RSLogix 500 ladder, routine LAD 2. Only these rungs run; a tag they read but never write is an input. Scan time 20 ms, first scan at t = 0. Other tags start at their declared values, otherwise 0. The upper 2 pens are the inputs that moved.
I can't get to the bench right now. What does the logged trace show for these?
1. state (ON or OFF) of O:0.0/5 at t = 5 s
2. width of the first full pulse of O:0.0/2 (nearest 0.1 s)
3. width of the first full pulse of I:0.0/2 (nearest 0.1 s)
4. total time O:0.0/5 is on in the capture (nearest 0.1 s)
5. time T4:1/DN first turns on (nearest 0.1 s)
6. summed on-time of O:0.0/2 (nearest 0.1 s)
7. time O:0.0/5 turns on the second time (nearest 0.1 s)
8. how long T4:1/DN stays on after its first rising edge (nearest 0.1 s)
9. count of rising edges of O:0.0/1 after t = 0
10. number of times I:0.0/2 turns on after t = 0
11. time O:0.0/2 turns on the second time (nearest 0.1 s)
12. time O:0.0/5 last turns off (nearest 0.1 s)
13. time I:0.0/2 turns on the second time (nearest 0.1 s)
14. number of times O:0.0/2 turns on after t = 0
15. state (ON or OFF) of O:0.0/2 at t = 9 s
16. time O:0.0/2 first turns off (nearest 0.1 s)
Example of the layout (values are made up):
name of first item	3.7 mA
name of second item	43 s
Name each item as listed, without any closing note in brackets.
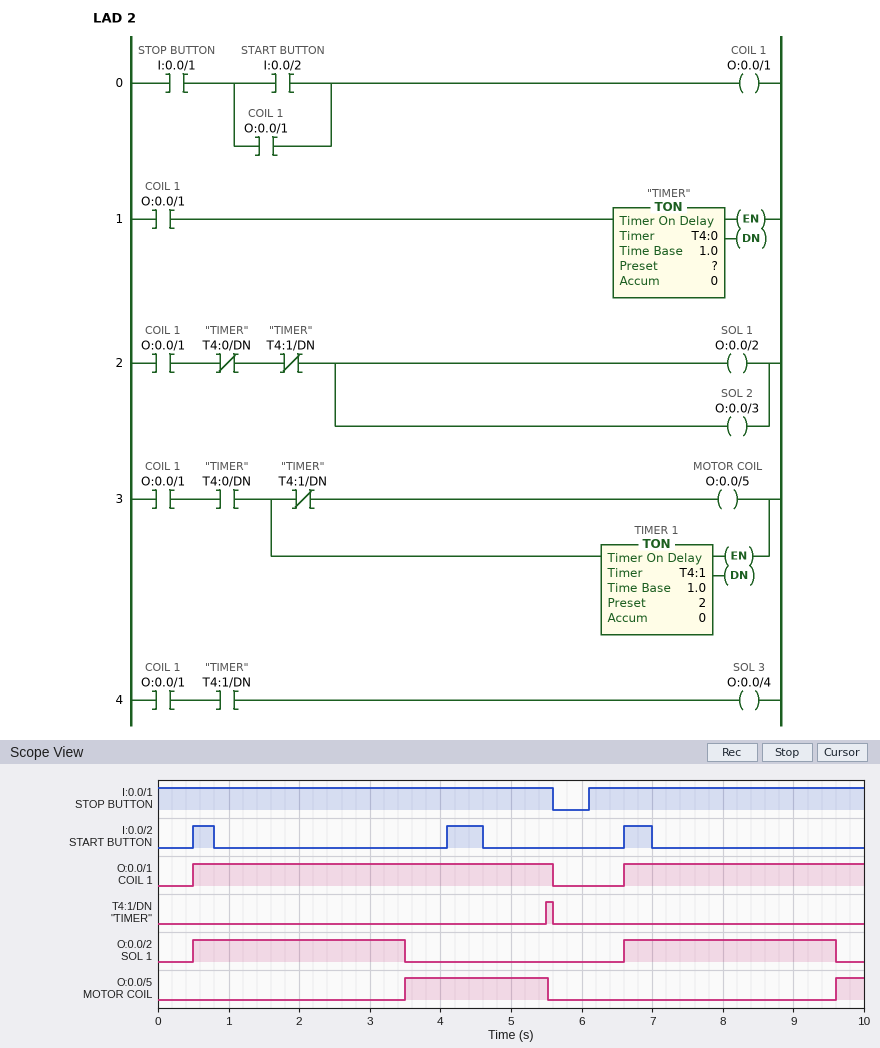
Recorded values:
state (ON or OFF) of O:0.0/5 at t = 5 s	ON
width of the first full pulse of O:0.0/2	3.0 s
width of the first full pulse of I:0.0/2	0.3 s
total time O:0.0/5 is on in the capture	2.4 s
time T4:1/DN first turns on	5.5 s
summed on-time of O:0.0/2	6.0 s
time O:0.0/5 turns on the second time	9.6 s
how long T4:1/DN stays on after its first rising edge	0.1 s
count of rising edges of O:0.0/1 after t = 0	2
number of times I:0.0/2 turns on after t = 0	3
time O:0.0/2 turns on the second time	6.6 s
time O:0.0/5 last turns off	5.5 s
time I:0.0/2 turns on the second time	4.1 s
number of times O:0.0/2 turns on after t = 0	2
state (ON or OFF) of O:0.0/2 at t = 9 s	ON
time O:0.0/2 first turns off	3.5 s
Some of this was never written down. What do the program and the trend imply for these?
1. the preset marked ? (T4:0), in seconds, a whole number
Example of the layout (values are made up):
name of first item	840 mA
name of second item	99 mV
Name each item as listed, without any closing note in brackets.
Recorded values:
the preset marked ? (T4:0), in seconds, a whole number	3 s
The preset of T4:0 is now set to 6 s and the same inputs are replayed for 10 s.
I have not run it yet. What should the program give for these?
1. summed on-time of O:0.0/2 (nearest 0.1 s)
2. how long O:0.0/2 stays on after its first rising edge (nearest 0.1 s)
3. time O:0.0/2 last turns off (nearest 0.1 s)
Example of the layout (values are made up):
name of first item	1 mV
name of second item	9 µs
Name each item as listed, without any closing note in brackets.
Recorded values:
summed on-time of O:0.0/2	8.5 s
how long O:0.0/2 stays on after its first rising edge	5.1 s
time O:0.0/2 last turns off	5.6 s
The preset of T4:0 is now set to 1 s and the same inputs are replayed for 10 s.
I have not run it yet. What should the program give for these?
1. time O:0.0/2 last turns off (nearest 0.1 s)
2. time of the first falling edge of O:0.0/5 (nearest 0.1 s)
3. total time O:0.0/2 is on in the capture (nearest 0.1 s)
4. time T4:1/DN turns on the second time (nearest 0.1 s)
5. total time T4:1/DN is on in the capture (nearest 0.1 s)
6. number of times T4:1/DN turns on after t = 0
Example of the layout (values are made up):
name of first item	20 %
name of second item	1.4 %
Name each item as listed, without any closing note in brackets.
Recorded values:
time O:0.0/2 last turns off	7.6 s
time of the first falling edge of O:0.0/5	3.5 s
total time O:0.0/2 is on in the capture	2.0 s
time T4:1/DN turns on the second time	9.6 s
total time T4:1/DN is on in the capture	2.5 s
number of times T4:1/DN turns on after t = 0	2
